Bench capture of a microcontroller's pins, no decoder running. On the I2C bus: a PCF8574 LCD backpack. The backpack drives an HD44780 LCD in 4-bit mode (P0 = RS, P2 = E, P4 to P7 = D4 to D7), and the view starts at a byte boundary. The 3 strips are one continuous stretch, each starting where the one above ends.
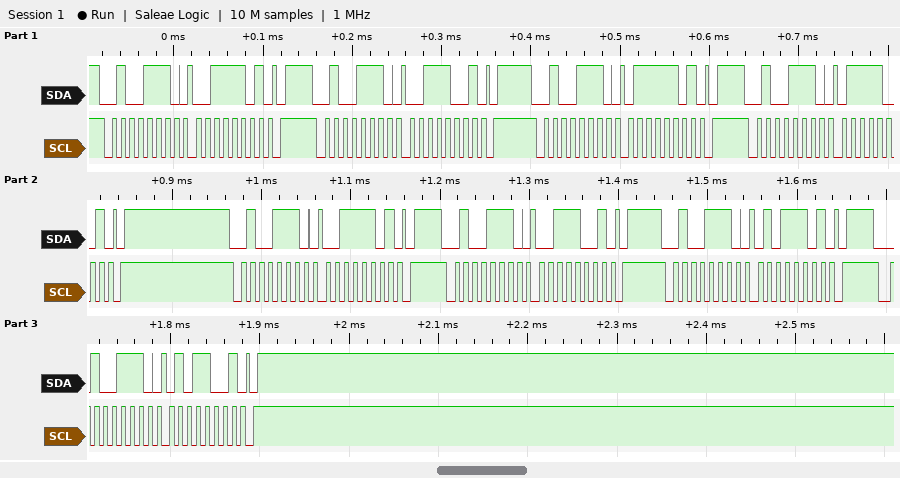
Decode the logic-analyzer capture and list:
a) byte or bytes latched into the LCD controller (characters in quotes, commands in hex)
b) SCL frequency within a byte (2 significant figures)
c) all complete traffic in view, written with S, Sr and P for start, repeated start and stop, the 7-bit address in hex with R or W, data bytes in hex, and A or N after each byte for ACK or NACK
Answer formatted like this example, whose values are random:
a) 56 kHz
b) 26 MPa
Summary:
a) '7' '5'
b) 100 kHz
c) S 27W A 3D A P S 27W A 39 A P S 27W A 7D A P S 27W A 79 A P S 27W A 3D A P S 27W A 39 A P S 27W A 5D A P S 27W A 59 A P
